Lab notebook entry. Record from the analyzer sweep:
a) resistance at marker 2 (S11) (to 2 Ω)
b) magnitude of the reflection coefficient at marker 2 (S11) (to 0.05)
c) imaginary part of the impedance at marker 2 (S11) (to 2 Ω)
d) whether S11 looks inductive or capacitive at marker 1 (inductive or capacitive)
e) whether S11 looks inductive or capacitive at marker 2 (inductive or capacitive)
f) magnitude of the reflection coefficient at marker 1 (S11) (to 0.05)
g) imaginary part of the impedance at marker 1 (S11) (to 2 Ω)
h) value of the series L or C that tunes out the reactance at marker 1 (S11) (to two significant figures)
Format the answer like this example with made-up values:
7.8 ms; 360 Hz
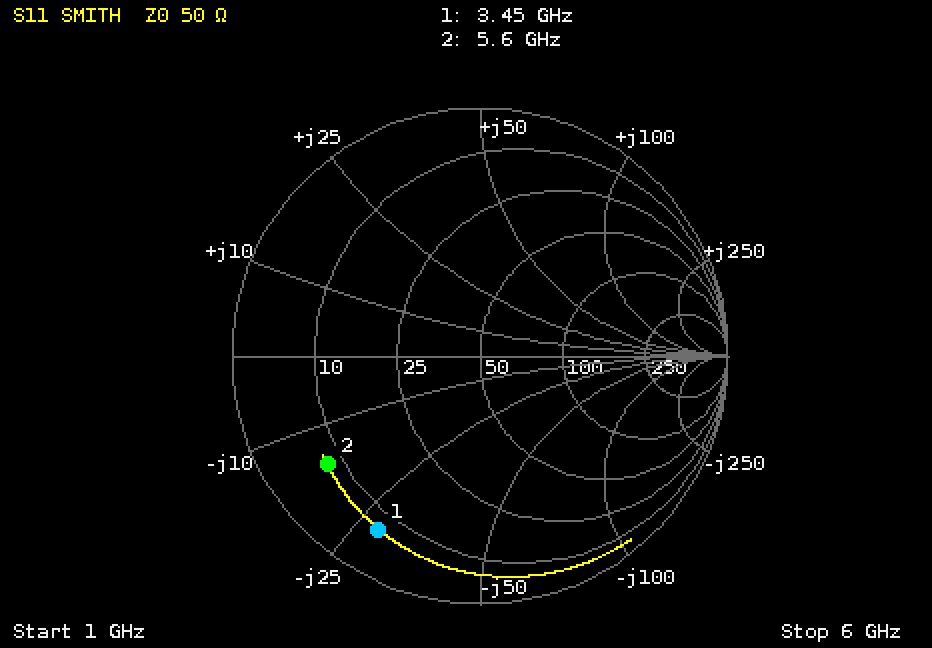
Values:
8 Ω; 0.75; -16 Ω; capacitive; capacitive; 0.80; -28 Ω; 1.3 nH
